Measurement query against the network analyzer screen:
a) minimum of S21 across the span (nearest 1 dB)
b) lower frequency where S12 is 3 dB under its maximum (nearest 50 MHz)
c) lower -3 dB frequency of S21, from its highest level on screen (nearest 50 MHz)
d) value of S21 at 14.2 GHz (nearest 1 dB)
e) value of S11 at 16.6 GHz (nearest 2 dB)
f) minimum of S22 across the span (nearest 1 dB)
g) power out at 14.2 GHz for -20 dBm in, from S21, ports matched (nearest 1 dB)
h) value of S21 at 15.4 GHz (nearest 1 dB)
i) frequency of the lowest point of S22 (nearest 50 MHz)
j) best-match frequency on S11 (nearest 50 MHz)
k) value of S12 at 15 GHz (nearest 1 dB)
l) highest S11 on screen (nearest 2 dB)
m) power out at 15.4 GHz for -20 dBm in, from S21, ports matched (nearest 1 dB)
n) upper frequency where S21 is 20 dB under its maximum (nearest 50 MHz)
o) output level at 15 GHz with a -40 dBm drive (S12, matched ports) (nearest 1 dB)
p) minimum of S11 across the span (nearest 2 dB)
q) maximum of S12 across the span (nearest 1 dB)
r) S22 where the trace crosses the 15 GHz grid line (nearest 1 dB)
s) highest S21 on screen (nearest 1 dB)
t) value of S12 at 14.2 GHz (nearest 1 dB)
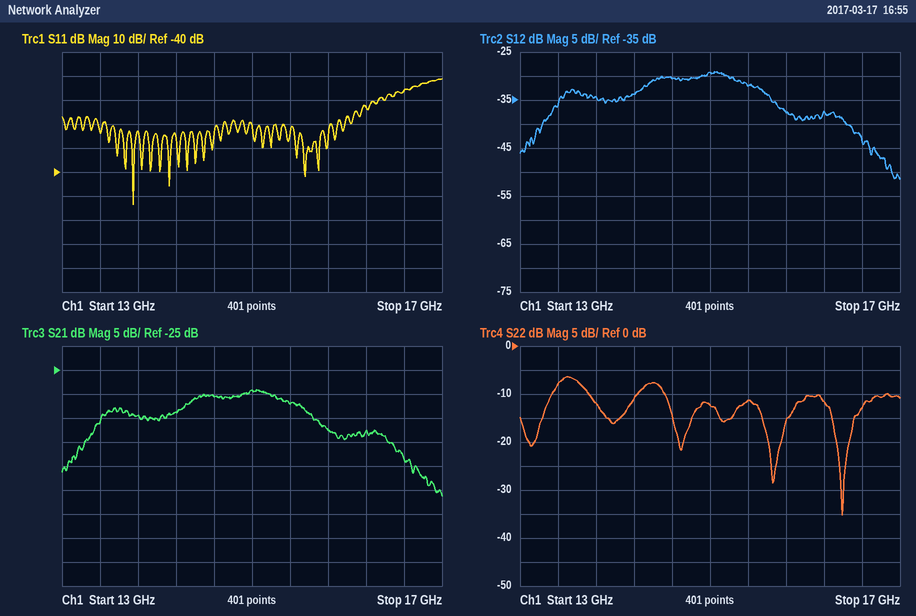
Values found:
-51 dB
14.35 GHz
14.30 GHz
-34 dB
-6 dB
-35 dB
-54 dBm
-32 dB
16.40 GHz
13.75 GHz
-29 dB
-2 dB
-52 dBm
16.90 GHz
-69 dBm
-54 dB
-29 dB
-12 dB
-29 dB
-34 dB
